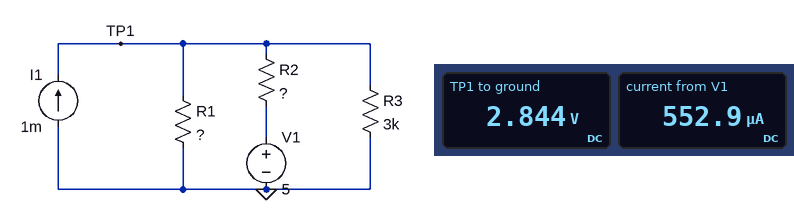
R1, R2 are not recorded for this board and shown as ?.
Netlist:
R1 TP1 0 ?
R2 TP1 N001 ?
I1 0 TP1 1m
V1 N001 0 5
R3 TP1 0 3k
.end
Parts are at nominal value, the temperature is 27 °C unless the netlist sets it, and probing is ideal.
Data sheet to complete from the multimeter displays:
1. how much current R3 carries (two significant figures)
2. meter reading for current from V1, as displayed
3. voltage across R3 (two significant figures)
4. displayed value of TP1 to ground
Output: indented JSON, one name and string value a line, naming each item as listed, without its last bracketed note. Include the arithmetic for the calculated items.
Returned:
{
  "how much current R3 carries": "(2.844 V) / 3 kΩ = 950 µA",
  "meter reading for current from V1, as displayed": "552.9 µA",
  "voltage across R3": "2.844 V = 2.8 V",
  "displayed value of TP1 to ground": "2.844 V"
}
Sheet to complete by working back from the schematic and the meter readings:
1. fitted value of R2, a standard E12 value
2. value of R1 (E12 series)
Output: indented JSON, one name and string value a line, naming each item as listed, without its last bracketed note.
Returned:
{
  "fitted value of R2, a standard E12 value": "3.9 kΩ",
  "value of R1": "4.7 kΩ"
}
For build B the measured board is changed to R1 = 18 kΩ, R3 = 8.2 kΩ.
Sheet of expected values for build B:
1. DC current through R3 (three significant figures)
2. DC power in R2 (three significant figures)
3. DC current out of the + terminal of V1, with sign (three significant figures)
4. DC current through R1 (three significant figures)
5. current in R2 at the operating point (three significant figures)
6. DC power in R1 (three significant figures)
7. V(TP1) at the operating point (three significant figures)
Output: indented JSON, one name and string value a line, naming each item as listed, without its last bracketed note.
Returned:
{
  "DC current through R3": "641 µA",
  "DC power in R2": "17.2 µW",
  "DC current out of the + terminal of V1, with sign": "-66.5 µA",
  "DC current through R1": "292 µA",
  "current in R2 at the operating point": "66.5 µA",
  "DC power in R1": "1.54 mW",
  "V(TP1) at the operating point": "5.26 V"
}
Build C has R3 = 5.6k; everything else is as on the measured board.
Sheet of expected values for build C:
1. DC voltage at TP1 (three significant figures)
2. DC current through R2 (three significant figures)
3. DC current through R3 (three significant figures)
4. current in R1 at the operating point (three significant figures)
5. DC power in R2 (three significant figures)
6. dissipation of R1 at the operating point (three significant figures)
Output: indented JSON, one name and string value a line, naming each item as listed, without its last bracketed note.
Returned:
{
  "DC voltage at TP1": "3.52 V",
  "DC current through R2": "379 µA",
  "DC current through R3": "629 µA",
  "current in R1 at the operating point": "750 µA",
  "DC power in R2": "559 µW",
  "dissipation of R1 at the operating point": "2.64 mW"
}
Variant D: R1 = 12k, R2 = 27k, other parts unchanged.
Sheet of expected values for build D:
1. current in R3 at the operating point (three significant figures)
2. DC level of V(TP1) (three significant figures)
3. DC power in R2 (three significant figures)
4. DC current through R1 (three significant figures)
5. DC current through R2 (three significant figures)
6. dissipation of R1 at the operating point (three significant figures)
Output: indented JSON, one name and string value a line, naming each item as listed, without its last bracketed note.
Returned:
{
  "current in R3 at the operating point": "871 µA",
  "DC level of V(TP1)": "2.61 V",
  "DC power in R2": "211 µW",
  "DC current through R1": "218 µA",
  "DC current through R2": "88.4 µA",
  "dissipation of R1 at the operating point": "569 µW"
}
